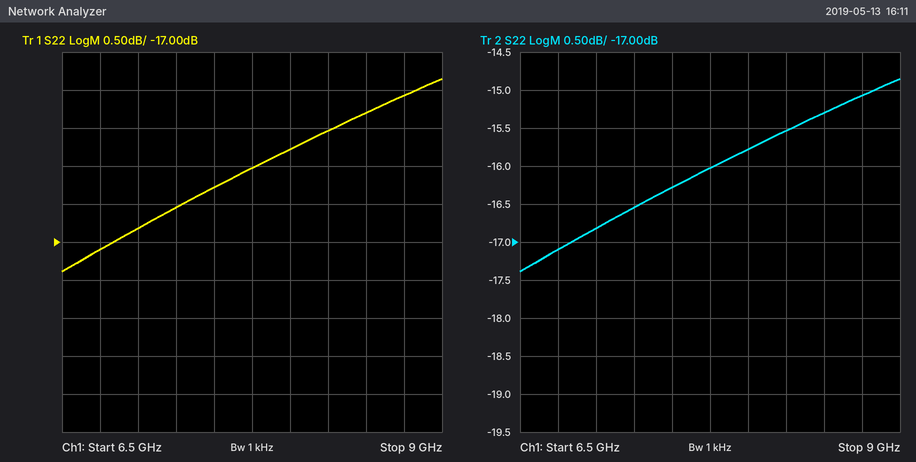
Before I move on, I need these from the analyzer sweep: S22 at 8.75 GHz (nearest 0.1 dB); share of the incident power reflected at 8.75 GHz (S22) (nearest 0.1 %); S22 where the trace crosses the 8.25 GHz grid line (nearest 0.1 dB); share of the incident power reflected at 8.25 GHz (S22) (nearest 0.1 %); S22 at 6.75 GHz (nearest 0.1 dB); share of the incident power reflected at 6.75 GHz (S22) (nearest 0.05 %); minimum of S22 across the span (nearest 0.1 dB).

-15.1 dB
3.1 %
-15.5 dB
2.8 %
-17.1 dB
1.95 %
-17.4 dB
